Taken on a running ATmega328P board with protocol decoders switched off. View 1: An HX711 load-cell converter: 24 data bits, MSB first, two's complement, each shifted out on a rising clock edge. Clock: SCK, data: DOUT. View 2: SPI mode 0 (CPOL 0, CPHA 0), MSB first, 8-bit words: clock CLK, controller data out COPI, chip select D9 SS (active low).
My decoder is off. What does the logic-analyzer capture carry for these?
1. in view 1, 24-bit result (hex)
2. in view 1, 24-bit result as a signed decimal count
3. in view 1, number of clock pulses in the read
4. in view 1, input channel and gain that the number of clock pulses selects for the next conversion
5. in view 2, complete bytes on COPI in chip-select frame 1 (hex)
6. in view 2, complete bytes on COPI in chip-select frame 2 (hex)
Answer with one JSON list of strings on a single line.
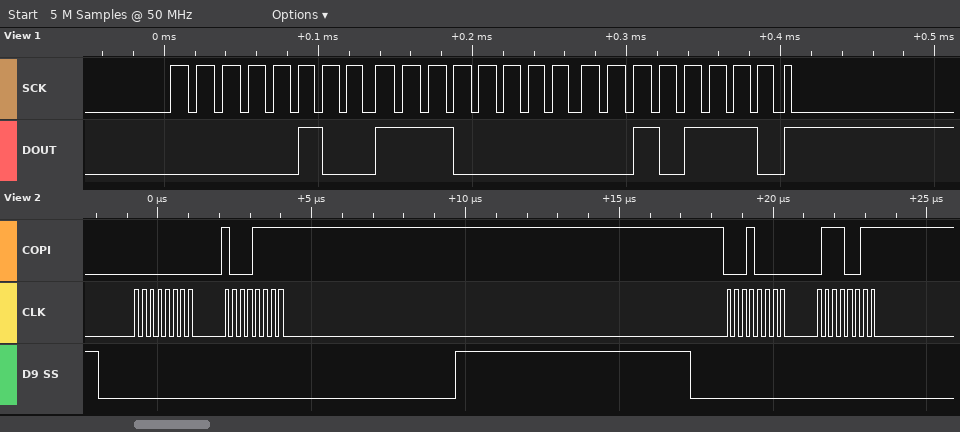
["0x04E02E", "319534", "25", "channel A, gain 128", "0x00 0x8F", "0x10 0x73"]
